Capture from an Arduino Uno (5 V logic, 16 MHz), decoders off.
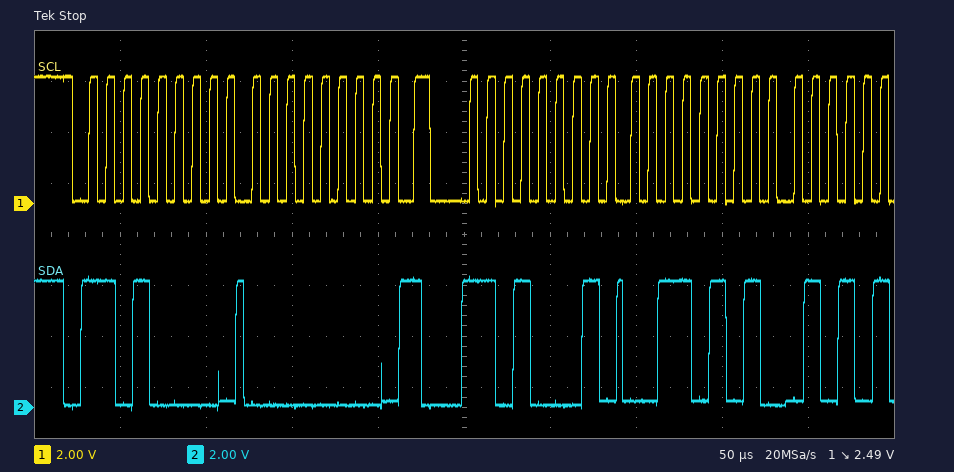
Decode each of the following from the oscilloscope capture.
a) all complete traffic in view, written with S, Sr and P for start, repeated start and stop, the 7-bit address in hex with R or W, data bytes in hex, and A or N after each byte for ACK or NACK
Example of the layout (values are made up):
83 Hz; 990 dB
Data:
S 68W A 00 A Sr 68R A 35 A
